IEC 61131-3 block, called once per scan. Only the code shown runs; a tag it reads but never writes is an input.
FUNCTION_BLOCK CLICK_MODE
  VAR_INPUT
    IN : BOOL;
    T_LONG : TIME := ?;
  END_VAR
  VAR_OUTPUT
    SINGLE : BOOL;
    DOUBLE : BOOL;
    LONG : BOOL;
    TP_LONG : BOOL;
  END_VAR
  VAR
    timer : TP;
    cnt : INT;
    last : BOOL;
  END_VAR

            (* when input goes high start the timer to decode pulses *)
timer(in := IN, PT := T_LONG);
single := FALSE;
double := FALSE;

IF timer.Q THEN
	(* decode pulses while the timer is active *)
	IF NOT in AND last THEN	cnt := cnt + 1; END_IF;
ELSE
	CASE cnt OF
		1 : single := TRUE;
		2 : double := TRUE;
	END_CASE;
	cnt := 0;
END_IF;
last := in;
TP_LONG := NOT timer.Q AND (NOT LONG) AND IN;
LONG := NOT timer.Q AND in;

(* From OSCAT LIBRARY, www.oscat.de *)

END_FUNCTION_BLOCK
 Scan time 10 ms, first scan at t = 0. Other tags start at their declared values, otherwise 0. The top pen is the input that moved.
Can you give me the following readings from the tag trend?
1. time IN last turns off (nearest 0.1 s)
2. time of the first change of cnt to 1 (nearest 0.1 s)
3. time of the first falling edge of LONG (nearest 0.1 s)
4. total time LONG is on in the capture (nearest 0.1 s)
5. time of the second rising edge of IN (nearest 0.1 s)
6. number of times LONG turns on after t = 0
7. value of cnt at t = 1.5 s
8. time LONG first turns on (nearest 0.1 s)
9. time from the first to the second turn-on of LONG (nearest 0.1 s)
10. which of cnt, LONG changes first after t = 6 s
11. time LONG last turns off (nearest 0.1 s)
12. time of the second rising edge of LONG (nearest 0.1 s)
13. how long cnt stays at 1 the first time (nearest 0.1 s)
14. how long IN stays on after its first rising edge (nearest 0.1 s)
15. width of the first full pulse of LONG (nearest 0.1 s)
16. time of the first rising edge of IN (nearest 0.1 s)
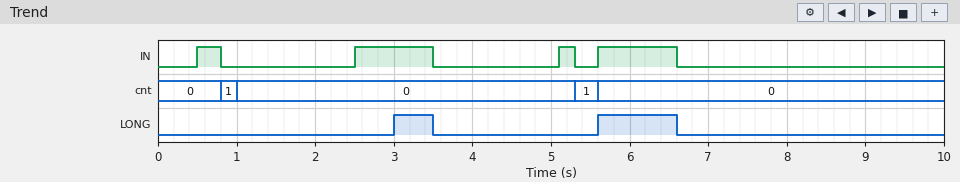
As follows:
6.6 s
0.8 s
3.5 s
1.5 s
2.5 s
2
0
3.0 s
2.6 s
LONG
6.6 s
5.6 s
0.2 s
0.3 s
0.5 s
0.5 s
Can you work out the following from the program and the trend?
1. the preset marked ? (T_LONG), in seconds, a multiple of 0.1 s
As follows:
0.5 s
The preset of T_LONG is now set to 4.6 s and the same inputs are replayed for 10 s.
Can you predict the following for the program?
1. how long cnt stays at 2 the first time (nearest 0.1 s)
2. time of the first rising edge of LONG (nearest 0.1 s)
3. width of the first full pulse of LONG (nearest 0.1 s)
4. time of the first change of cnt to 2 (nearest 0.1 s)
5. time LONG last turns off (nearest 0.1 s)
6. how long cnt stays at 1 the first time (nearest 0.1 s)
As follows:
1.6 s
5.1 s
0.2 s
3.5 s
5.3 s
2.7 s
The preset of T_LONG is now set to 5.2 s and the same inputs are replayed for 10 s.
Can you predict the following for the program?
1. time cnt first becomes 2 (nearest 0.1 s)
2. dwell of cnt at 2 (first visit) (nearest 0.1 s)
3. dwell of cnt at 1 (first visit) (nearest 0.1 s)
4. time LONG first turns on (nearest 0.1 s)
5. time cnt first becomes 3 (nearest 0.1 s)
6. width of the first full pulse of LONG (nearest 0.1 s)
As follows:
3.5 s
1.8 s
2.7 s
5.7 s
5.3 s
0.9 s
